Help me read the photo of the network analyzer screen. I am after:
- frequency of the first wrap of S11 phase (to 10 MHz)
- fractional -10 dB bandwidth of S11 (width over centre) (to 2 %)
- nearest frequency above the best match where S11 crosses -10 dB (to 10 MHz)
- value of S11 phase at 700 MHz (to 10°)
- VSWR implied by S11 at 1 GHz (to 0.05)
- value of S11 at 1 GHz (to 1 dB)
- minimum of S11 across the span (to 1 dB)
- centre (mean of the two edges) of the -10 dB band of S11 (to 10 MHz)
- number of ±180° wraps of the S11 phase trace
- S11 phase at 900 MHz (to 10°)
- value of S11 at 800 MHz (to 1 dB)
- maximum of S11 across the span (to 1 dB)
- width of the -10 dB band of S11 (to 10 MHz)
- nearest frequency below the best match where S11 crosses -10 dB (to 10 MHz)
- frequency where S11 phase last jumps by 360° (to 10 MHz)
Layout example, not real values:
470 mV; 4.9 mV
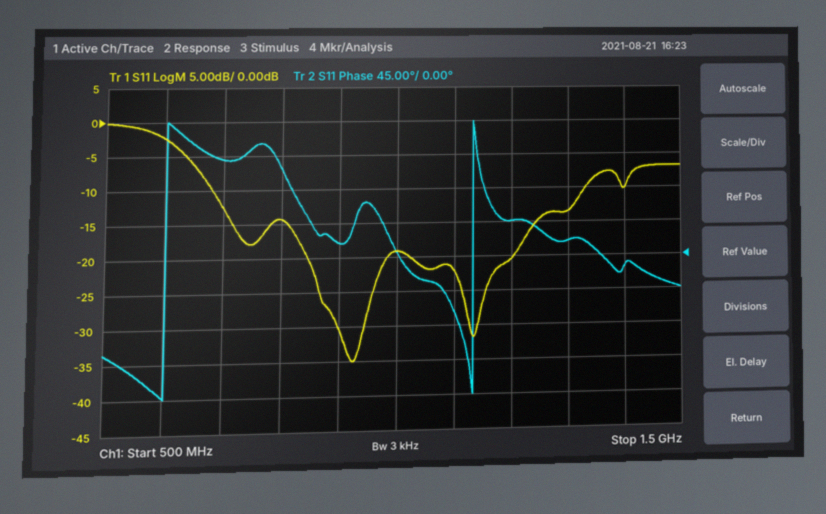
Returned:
600 MHz; 64 %; 1.33 GHz; 130°; 1.25; -19 dB; -35 dB; 1.01 GHz; 2; 20°; -14 dB; 0 dB; 650 MHz; 680 MHz; 1.13 GHz
